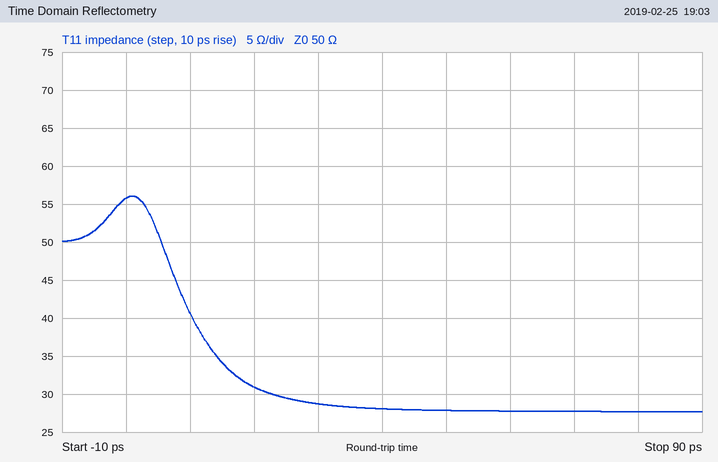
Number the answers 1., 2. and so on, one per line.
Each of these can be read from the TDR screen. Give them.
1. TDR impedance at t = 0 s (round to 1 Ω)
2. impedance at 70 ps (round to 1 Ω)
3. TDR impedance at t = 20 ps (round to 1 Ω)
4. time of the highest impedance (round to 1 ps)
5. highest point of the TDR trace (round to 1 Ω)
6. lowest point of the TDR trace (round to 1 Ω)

1. 56 Ω
2. 28 Ω
3. 31 Ω
4. 1 ps
5. 56 Ω
6. 28 Ω
